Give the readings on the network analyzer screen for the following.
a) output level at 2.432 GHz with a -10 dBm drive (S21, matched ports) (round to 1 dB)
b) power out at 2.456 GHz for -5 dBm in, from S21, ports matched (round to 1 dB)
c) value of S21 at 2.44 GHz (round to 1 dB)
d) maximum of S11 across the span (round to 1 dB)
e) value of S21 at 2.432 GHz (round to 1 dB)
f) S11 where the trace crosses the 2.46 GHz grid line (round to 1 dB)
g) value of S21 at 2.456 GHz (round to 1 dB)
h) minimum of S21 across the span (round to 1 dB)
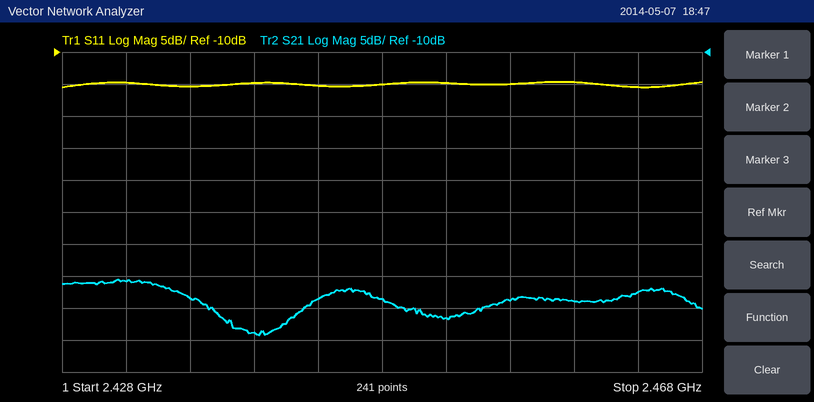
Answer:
-56 dBm
-54 dBm
-54 dB
-15 dB
-46 dB
-15 dB
-49 dB
-54 dB
